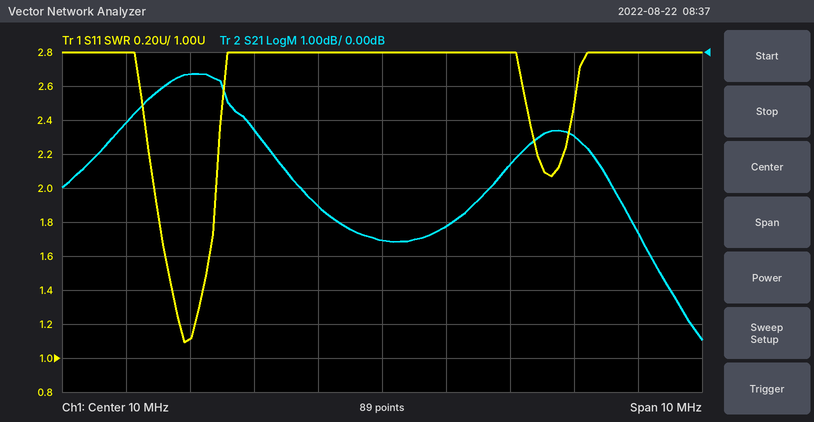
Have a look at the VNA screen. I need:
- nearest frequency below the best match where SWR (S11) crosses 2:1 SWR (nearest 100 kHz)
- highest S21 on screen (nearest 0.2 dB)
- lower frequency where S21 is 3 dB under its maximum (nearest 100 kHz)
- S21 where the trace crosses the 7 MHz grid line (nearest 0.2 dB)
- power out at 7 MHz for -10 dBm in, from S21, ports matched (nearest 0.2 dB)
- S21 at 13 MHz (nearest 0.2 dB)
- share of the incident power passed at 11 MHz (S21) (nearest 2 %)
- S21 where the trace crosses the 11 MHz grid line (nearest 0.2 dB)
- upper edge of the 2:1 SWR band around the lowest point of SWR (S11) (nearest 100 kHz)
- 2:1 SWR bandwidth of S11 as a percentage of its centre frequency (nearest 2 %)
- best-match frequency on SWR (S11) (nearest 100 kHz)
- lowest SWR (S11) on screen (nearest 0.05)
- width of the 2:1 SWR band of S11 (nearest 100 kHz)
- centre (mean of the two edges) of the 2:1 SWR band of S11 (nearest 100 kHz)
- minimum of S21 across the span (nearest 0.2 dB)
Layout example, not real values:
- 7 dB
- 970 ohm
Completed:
- 6.4 MHz
- -0.6 dB
- 5.2 MHz
- -0.6 dB
- -10.6 dBm
- -2.4 dB
- 30 %
- -5.2 dB
- 7.4 MHz
- 14 %
- 6.9 MHz
- 1.10
- 1.0 MHz
- 6.9 MHz
- -8.4 dB
